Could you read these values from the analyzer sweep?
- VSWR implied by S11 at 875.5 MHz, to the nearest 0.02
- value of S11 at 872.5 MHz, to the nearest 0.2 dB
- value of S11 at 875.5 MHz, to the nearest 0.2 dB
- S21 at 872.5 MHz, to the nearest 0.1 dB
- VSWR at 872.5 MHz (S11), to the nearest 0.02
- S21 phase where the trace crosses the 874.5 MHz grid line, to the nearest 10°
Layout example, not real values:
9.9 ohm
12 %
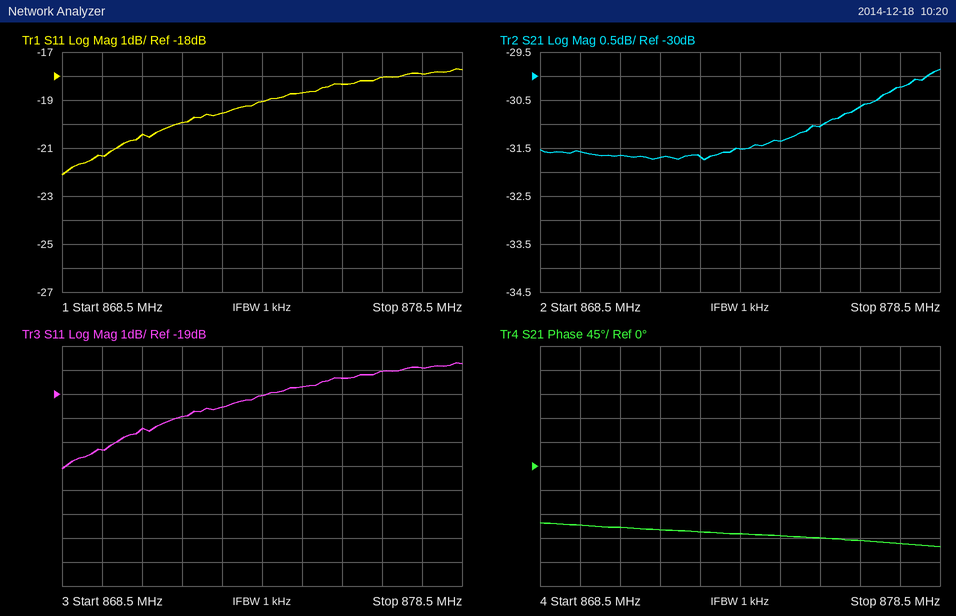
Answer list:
1.28
-19.6 dB
-18.4 dB
-31.7 dB
1.24
-130°
